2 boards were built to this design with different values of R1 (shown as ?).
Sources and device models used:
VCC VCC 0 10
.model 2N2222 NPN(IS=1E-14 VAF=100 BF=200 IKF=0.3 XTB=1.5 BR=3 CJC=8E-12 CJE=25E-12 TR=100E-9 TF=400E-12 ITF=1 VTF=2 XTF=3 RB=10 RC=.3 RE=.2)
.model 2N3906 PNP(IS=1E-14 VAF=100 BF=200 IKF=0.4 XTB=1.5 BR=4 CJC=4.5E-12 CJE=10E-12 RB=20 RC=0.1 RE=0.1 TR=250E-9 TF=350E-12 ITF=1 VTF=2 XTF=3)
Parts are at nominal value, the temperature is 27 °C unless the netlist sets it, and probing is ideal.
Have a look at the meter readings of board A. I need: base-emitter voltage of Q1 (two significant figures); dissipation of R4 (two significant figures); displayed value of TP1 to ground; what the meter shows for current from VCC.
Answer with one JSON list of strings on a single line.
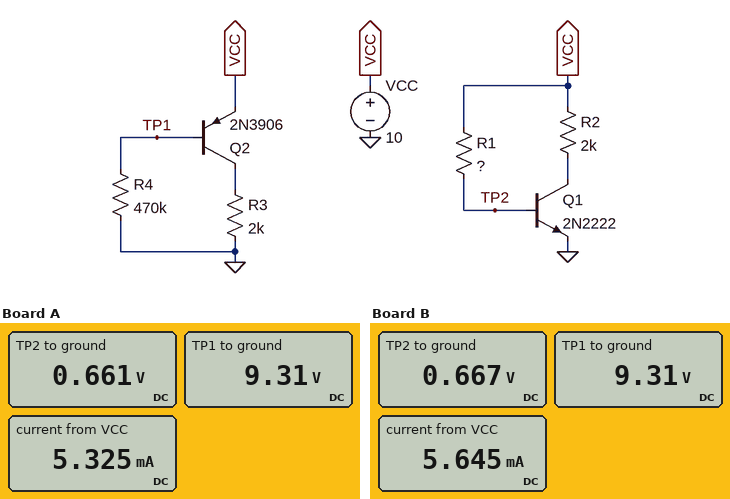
["660 mV", "180 µW", "9.31 V", "5.325 mA"]
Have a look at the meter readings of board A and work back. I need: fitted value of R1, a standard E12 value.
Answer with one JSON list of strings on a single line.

["1.5 MΩ"]
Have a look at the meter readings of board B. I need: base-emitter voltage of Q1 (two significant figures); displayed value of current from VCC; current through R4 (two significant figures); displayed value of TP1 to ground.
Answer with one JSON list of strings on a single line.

["670 mV", "5.645 mA", "20 µA", "9.31 V"]
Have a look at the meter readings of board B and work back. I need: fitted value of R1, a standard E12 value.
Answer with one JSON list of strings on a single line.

["1.2 MΩ"]
